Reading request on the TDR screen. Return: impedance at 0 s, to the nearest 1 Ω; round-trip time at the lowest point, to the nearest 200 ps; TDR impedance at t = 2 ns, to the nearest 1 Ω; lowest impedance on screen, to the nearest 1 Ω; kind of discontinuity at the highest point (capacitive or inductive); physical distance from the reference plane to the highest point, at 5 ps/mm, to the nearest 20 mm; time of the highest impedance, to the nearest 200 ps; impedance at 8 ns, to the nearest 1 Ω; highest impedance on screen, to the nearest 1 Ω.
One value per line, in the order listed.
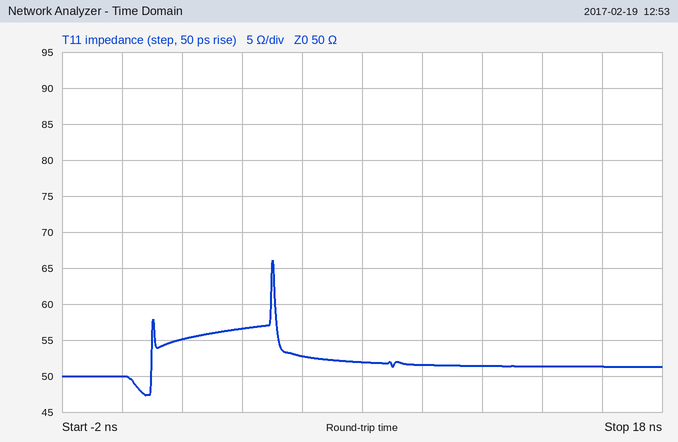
50 Ω
800 ps
55 Ω
47 Ω
inductive
500 mm
5.0 ns
52 Ω
66 Ω
